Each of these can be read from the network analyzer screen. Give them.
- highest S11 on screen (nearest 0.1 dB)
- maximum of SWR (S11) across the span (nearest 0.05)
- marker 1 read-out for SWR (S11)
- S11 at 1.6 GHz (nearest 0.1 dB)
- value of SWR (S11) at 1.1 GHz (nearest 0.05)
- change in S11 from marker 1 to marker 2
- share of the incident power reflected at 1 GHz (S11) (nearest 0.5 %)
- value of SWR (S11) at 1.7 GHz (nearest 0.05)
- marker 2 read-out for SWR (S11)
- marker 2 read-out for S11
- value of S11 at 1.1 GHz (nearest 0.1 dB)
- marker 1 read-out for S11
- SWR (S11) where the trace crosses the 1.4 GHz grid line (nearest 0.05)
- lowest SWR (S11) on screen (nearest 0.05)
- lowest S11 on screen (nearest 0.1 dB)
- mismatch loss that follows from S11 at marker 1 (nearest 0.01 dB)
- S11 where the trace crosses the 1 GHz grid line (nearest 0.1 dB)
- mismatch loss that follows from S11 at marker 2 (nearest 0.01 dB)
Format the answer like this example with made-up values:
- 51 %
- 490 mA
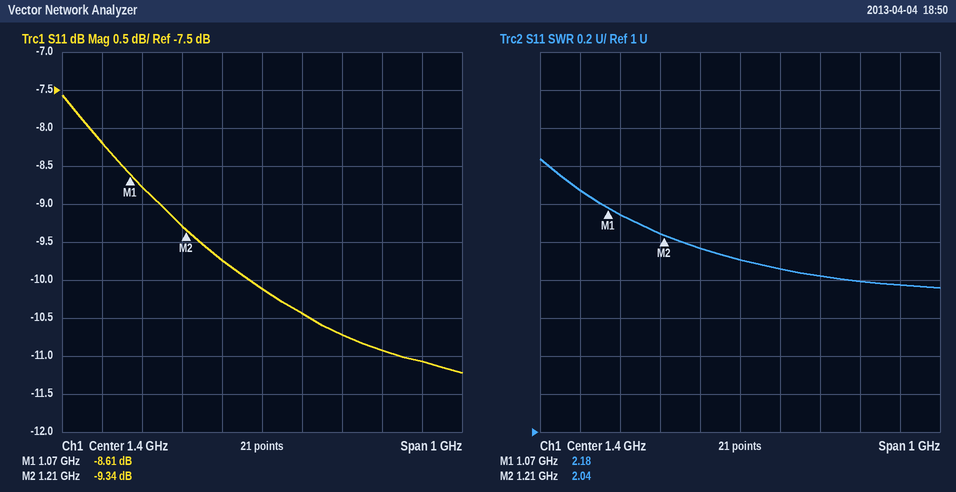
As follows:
- -7.6 dB
- 2.45
- 2.18
- -10.7 dB
- 2.15
- -0.73 dB
- 15.0 %
- 1.80
- 2.04
- -9.34 dB
- -8.8 dB
- -8.61 dB
- 1.90
- 1.75
- -11.2 dB
- 0.64 dB
- -8.2 dB
- 0.54 dB
